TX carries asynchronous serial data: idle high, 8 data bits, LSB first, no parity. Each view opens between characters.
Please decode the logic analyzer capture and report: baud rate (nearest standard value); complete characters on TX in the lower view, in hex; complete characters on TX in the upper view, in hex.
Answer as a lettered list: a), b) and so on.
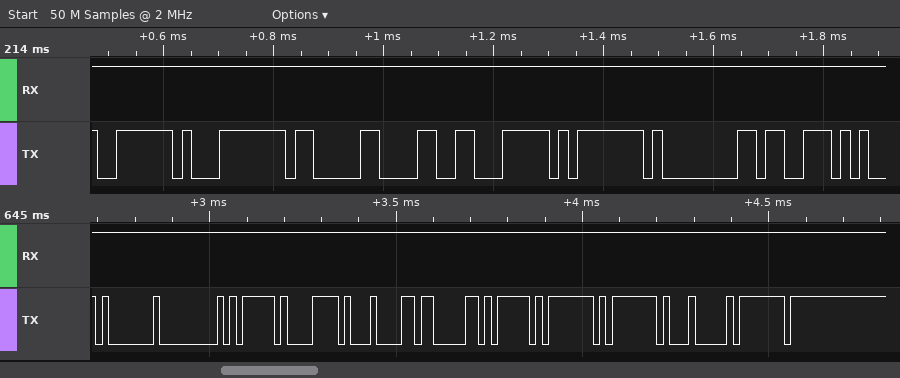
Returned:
a) 57600 baud
b) 01, 00, 7D, 78, 84, 83, 7D, 7F, 7F, 04, 7F
c) 7E, FC, 83, 98, 7C, 7F, 80, 73
